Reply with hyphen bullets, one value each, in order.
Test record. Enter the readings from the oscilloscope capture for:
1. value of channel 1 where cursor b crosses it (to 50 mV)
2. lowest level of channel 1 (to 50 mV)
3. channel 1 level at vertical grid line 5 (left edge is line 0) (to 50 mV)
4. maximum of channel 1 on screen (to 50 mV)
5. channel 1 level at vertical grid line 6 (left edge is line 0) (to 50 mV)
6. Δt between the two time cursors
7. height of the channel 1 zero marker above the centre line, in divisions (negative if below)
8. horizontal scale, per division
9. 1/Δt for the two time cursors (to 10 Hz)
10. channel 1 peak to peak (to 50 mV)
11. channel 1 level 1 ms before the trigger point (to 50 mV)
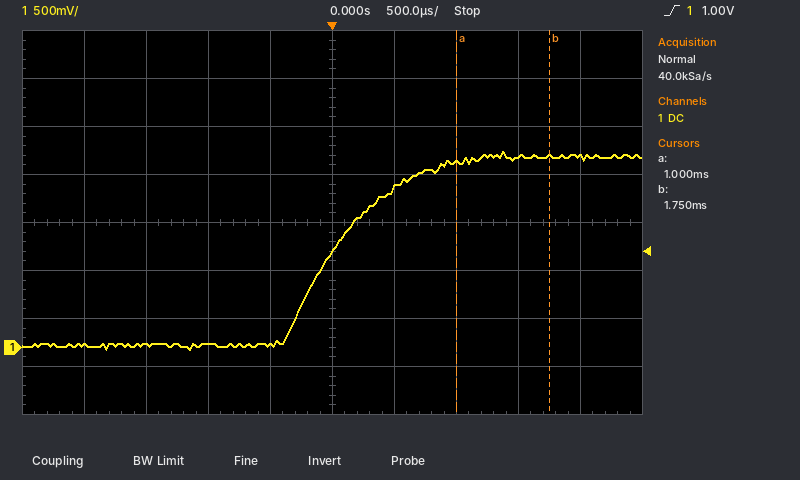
- 2.00 V
- 0 mV
- 1.00 V
- 2.05 V
- 1.65 V
- 750 µs
- -2.6 div
- 500 µs
- 1.33 kHz
- 2.05 V
- 50 mV
